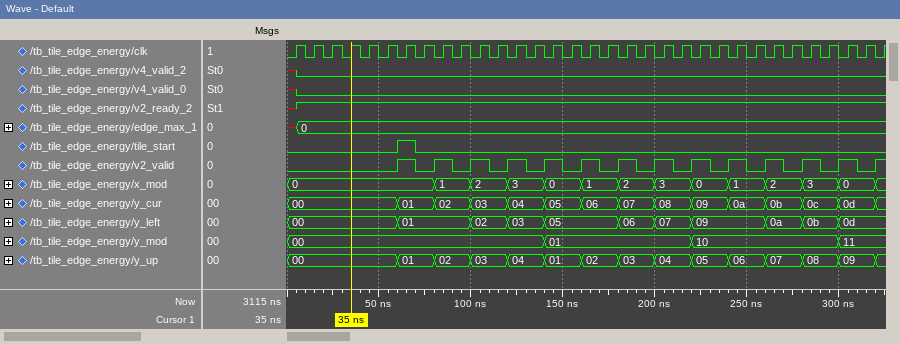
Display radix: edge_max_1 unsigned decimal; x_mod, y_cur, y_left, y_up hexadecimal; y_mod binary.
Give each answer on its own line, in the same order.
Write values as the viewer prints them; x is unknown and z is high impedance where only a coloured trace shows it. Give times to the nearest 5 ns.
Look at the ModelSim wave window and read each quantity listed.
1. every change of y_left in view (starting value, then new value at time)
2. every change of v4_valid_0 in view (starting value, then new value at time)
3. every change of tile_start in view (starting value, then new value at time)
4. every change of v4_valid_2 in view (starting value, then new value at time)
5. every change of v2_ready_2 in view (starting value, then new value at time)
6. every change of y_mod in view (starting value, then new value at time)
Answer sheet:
00, 01 at 60 ns, 02 at 100 ns, 03 at 120 ns, 05 at 140 ns, 06 at 180 ns, 07 at 200 ns, 09 at 220 ns, 0a at 260 ns, 0b at 280 ns, 0d at 300 ns
x, 0 at 5 ns
0, 1 at 60 ns, 0 at 70 ns
x, 0 at 5 ns
x, 1 at 5 ns
00, 01 at 140 ns, 10 at 220 ns, 11 at 300 ns
